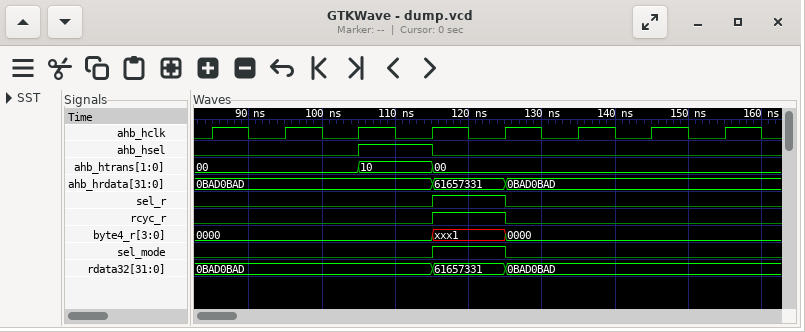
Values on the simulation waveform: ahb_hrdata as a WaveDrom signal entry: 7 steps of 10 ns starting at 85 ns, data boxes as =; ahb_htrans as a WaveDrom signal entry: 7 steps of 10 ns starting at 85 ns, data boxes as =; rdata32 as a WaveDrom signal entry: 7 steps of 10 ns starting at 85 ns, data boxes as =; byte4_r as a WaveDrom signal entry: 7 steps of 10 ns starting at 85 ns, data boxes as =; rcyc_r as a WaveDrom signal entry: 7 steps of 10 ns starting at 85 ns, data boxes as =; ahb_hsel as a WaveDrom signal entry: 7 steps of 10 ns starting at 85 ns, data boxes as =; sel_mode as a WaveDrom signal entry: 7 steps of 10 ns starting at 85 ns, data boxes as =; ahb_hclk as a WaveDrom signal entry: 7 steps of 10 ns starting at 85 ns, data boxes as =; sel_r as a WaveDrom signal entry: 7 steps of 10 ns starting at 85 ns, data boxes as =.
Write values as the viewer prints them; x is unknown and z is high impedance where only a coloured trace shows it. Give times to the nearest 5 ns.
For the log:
{name: 'ahb_hrdata', wave: '=..==..', data: '0BAD0BAD 61657331 0BAD0BAD'}
{name: 'ahb_htrans', wave: '=.==...', data: '00 10 00'}
{name: 'rdata32', wave: '=..==..', data: '0BAD0BAD 61657331 0BAD0BAD'}
{name: 'byte4_r', wave: '=..==..', data: '0000 xxx1 0000'}
{name: 'rcyc_r', wave: '0..10..'}
{name: 'ahb_hsel', wave: '0.10...'}
{name: 'sel_mode', wave: '0..10..'}
{name: 'ahb_hclk', wave: 'p......'}
{name: 'sel_r', wave: '0..10..'}
